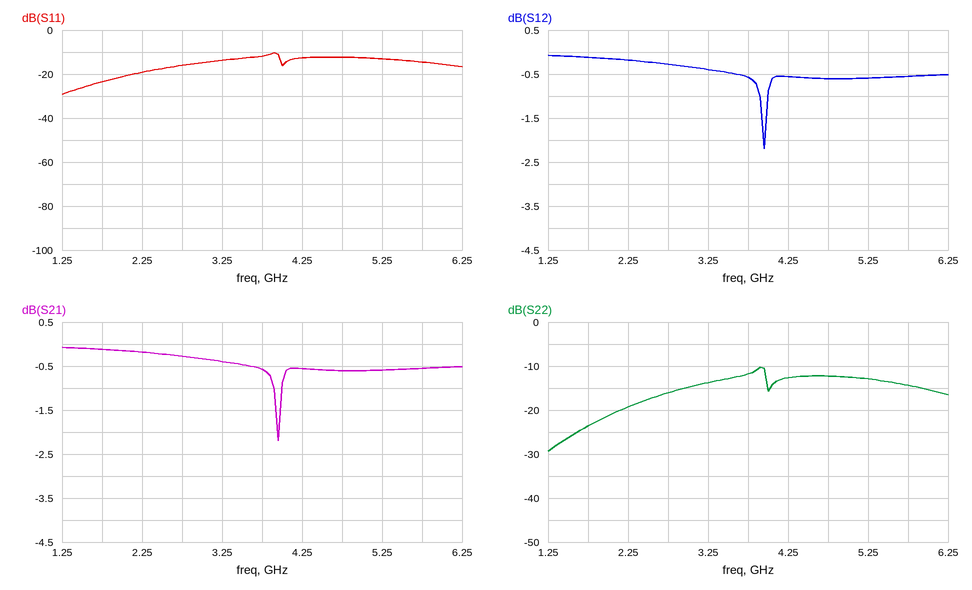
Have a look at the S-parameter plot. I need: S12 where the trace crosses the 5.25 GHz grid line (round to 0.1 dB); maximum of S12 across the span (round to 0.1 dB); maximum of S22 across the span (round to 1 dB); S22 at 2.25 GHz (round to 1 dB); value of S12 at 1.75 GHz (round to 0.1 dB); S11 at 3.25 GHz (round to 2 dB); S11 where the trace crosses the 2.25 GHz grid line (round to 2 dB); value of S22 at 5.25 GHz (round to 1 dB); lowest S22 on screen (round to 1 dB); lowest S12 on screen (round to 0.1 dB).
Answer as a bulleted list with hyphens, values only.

- -0.6 dB
- -0.1 dB
- -10 dB
- -19 dB
- -0.1 dB
- -14 dB
- -20 dB
- -13 dB
- -29 dB
- -2.2 dB
